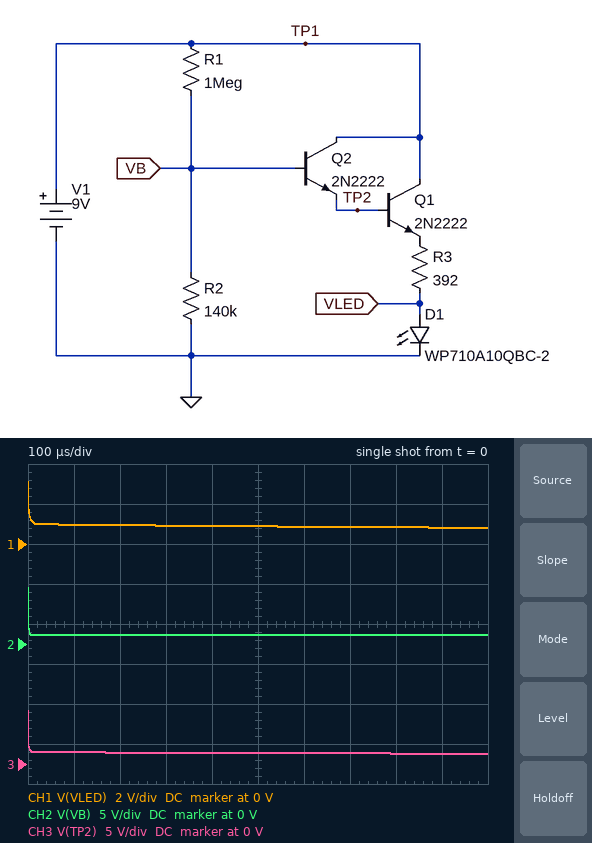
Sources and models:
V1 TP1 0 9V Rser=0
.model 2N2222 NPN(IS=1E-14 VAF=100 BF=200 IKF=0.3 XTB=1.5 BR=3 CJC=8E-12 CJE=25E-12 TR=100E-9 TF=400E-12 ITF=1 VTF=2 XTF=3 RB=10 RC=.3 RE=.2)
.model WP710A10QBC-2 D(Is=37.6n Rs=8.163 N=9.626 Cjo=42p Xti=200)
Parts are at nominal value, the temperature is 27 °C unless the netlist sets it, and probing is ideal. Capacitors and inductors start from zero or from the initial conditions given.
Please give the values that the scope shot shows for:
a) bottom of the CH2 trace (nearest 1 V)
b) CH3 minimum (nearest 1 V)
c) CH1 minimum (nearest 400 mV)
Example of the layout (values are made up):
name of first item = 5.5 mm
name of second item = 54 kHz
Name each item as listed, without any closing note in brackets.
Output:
bottom of the CH2 trace = 1 V
CH3 minimum = 1 V
CH1 minimum = 800 mV
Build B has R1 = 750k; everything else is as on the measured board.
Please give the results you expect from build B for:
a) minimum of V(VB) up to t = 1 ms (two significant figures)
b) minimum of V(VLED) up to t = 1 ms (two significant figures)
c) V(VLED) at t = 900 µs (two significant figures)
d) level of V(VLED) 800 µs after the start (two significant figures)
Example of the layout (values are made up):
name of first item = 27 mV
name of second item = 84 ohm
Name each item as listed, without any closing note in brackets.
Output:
minimum of V(VB) up to t = 1 ms = 1.4 V
minimum of V(VLED) up to t = 1 ms = 890 mV
V(VLED) at t = 900 µs = 910 mV
level of V(VLED) 800 µs after the start = 930 mV
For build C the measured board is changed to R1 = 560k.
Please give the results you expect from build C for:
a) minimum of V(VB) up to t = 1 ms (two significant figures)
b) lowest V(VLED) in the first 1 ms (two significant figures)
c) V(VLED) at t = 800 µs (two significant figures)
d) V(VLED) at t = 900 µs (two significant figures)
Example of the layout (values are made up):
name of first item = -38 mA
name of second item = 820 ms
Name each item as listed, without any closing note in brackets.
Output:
minimum of V(VB) up to t = 1 ms = 1.8 V
lowest V(VLED) in the first 1 ms = 980 mV
V(VLED) at t = 800 µs = 1.0 V
V(VLED) at t = 900 µs = 990 mV
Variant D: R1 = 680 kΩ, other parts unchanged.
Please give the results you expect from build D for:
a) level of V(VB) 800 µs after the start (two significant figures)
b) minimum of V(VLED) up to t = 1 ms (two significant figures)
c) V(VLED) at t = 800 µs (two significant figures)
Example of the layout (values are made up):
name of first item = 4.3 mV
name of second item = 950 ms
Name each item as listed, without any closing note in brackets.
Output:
level of V(VB) 800 µs after the start = 1.5 V
minimum of V(VLED) up to t = 1 ms = 920 mV
V(VLED) at t = 800 µs = 960 mV
